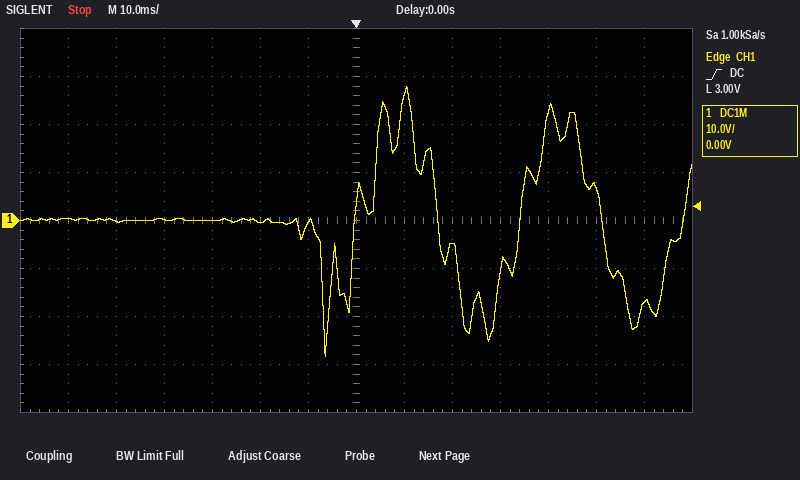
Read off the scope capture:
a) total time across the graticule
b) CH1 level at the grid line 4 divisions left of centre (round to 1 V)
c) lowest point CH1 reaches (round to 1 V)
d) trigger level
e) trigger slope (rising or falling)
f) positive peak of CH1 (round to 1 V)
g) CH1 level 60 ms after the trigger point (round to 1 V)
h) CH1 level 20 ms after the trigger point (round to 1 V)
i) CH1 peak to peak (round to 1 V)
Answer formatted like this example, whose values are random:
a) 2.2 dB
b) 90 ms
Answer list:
a) 140 ms
b) 0 V
c) -28 V
d) 3.00 V
e) rising
f) 28 V
g) -17 V
h) -5 V
i) 56 V
